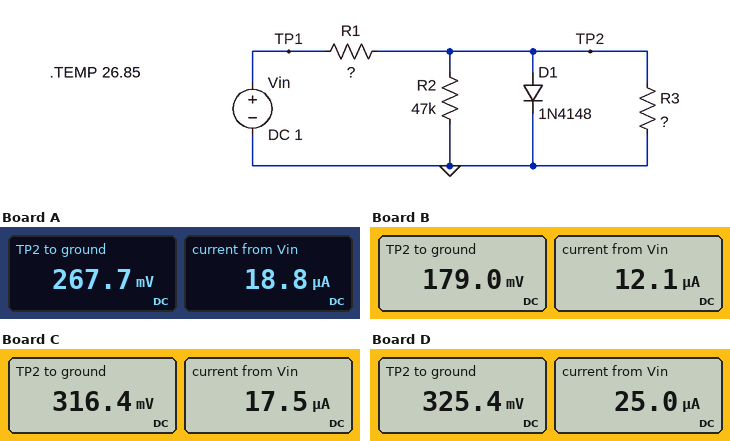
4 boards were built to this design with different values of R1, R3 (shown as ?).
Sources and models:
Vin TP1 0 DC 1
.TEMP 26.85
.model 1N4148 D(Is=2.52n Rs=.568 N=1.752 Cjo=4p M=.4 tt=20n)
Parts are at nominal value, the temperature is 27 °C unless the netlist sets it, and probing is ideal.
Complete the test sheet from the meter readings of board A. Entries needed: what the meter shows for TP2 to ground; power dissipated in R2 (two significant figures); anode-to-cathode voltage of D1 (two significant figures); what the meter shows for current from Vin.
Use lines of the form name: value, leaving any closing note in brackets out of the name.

what the meter shows for TP2 to ground: 267.7 mV
power dissipated in R2: 1.5 µW
anode-to-cathode voltage of D1: 270 mV
what the meter shows for current from Vin: 18.8 µA
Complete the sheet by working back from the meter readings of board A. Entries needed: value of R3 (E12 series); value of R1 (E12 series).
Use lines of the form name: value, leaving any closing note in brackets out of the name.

value of R3: 22 kΩ
value of R1: 39 kΩ
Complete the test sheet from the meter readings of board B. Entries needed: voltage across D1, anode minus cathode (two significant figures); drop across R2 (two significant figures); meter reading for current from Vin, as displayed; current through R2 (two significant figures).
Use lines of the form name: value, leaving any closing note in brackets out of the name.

voltage across D1, anode minus cathode: 180 mV
drop across R2: 180 mV
meter reading for current from Vin, as displayed: 12.1 µA
current through R2: 3.8 µA
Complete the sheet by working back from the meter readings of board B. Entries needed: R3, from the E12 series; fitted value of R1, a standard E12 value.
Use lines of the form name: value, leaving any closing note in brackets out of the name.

R3, from the E12 series: 22 kΩ
fitted value of R1, a standard E12 value: 68 kΩ
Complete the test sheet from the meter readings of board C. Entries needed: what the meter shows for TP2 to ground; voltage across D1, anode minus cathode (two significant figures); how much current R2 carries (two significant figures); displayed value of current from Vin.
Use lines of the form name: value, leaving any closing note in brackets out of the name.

what the meter shows for TP2 to ground: 316.4 mV
voltage across D1, anode minus cathode: 320 mV
how much current R2 carries: 6.7 µA
displayed value of current from Vin: 17.5 µA
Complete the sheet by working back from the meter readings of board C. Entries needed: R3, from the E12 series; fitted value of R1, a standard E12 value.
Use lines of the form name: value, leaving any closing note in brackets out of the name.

R3, from the E12 series: 39 kΩ
fitted value of R1, a standard E12 value: 39 kΩ
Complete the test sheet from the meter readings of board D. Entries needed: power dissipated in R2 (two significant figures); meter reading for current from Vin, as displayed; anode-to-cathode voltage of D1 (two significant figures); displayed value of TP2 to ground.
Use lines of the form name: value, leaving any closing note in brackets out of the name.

power dissipated in R2: 2.3 µW
meter reading for current from Vin, as displayed: 25.0 µA
anode-to-cathode voltage of D1: 330 mV
displayed value of TP2 to ground: 325.4 mV
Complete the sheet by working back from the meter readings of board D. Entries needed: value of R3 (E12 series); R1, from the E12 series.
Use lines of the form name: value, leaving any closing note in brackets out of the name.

value of R3: 22 kΩ
R1, from the E12 series: 27 kΩ
